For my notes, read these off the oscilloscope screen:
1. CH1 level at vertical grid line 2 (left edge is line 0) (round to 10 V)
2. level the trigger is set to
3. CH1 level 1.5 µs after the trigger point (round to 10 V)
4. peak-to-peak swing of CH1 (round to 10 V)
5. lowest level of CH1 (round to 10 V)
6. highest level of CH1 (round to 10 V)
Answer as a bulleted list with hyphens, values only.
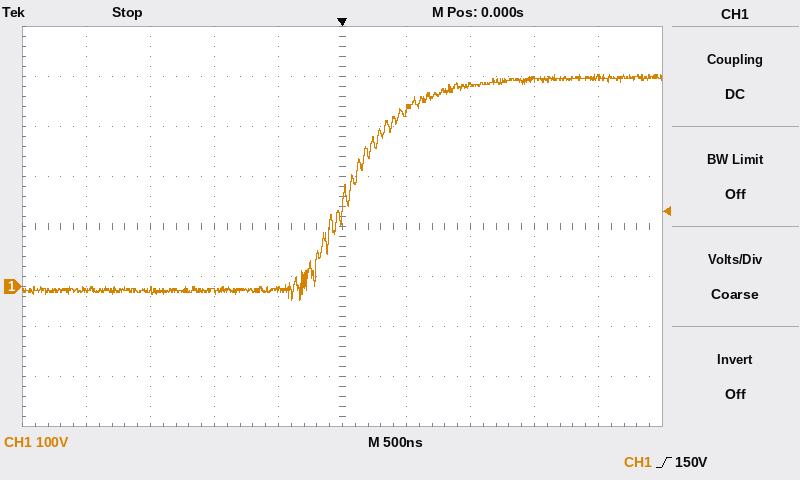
- -10 V
- 150 V
- 410 V
- 450 V
- -30 V
- 420 V
